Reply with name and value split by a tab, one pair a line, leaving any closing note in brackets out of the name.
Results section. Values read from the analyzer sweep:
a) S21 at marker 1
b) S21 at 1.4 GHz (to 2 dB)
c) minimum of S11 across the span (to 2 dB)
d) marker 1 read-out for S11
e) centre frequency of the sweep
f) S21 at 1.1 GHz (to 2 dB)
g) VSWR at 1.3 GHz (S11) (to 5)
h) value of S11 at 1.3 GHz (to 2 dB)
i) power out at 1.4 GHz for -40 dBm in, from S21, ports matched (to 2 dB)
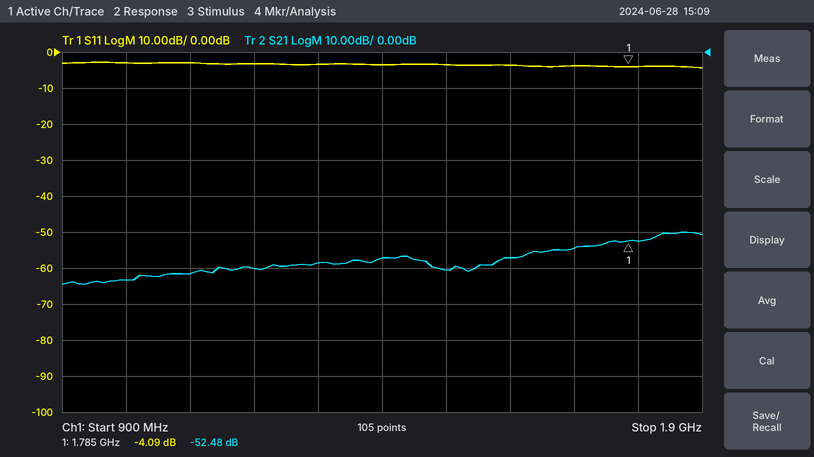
S21 at marker 1	-52.48 dB
S21 at 1.4 GHz	-58 dB
minimum of S11 across the span	-4 dB
marker 1 read-out for S11	-4.09 dB
centre frequency of the sweep	1.4 GHz
S21 at 1.1 GHz	-62 dB
VSWR at 1.3 GHz (S11)	5
value of S11 at 1.3 GHz	-4 dB
power out at 1.4 GHz for -40 dBm in, from S21, ports matched	-98 dBm
